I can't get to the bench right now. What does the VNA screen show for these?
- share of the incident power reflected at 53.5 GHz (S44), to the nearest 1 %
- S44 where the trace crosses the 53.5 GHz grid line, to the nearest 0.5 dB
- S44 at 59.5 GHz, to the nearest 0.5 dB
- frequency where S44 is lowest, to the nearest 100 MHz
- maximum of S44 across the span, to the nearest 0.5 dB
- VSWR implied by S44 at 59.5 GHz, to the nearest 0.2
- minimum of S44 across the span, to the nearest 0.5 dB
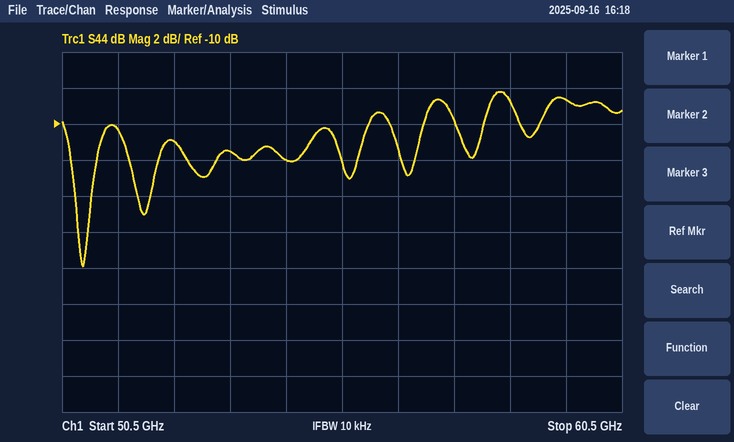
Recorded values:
7 %
-11.5 dB
-8.5 dB
50.9 GHz
-8.0 dB
2.2
-18.0 dB
